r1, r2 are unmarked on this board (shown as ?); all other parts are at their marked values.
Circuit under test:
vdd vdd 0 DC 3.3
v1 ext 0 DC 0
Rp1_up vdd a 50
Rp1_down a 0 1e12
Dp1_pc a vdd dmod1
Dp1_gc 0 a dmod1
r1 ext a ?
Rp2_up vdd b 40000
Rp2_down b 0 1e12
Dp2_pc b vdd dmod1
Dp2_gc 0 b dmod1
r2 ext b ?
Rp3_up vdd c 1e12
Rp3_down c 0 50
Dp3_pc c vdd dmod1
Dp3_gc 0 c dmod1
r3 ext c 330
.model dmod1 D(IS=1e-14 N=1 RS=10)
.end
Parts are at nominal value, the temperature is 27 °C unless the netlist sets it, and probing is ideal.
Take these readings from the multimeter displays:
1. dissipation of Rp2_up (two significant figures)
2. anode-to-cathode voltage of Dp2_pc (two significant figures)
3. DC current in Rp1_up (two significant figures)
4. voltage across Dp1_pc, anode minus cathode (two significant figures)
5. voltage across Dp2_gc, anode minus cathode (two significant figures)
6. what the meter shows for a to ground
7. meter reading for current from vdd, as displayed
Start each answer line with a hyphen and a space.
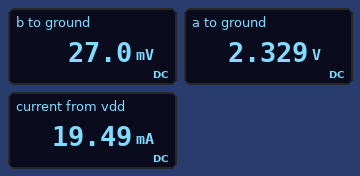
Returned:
- 270 µW
- -3.3 V
- 19 mA
- -970 mV
- -27 mV
- 2.329 V
- 19.49 mA
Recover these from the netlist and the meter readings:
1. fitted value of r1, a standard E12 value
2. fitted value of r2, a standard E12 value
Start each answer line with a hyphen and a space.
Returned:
- 120 Ω
- 330 Ω
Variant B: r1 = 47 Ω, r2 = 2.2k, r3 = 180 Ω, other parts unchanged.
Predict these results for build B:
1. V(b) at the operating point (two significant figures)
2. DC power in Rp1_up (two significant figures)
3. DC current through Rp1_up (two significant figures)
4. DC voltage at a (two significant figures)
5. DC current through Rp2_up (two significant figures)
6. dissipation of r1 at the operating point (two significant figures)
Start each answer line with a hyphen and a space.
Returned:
- 170 mV
- 58 mW
- 34 mA
- 1.6 V
- 78 µA
- 54 mW
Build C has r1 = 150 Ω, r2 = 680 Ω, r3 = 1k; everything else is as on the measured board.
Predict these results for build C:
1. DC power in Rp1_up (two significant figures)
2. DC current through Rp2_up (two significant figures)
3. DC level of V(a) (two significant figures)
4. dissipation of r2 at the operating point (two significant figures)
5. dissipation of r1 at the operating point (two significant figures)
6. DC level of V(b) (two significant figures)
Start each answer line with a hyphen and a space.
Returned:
- 14 mW
- 81 µA
- 2.5 V
- 4.5 µW
- 41 mW
- 55 mV
